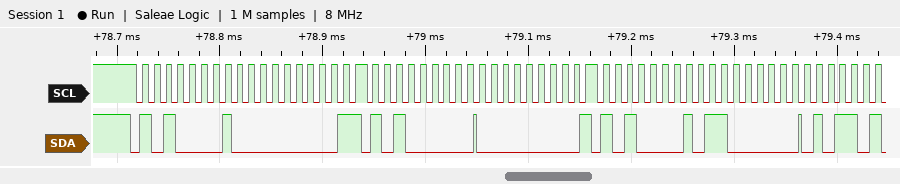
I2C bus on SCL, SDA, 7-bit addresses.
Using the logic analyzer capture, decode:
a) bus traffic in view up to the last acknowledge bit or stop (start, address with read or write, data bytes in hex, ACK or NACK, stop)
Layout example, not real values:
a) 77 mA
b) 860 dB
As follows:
a) start, address 50 read ACK, 00 NACK, repeated start, address 50 write ACK, 00 ACK, repeated start, address 50 read ACK, C0 ACK
